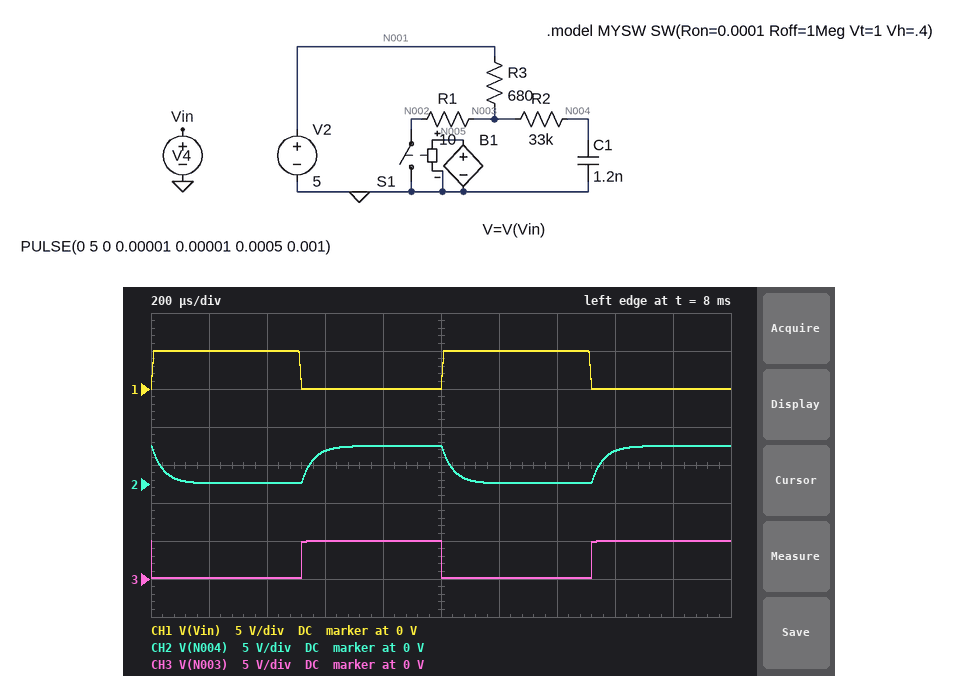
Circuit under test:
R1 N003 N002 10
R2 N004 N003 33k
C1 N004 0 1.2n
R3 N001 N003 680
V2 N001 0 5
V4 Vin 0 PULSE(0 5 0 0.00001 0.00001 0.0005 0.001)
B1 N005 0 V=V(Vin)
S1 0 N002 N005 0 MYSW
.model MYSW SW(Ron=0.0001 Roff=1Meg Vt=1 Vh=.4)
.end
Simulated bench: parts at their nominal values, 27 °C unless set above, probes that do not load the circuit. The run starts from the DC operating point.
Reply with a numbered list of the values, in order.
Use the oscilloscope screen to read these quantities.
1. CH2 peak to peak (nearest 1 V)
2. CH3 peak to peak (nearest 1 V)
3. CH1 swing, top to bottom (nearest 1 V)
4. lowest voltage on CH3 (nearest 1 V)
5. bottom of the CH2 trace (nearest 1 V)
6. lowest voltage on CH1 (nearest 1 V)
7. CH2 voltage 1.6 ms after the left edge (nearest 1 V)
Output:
1. 5 V
2. 5 V
3. 5 V
4. 0 V
5. 0 V
6. 0 V
7. 4 V
